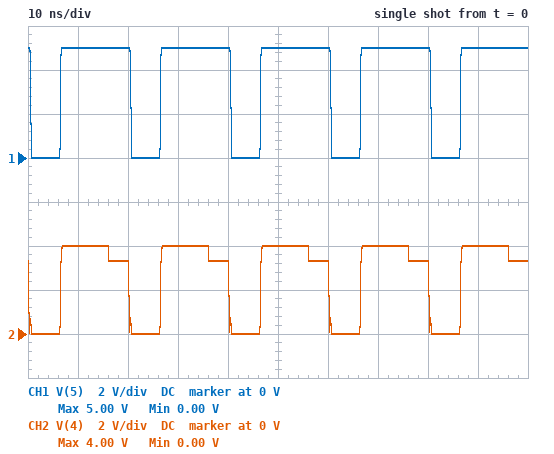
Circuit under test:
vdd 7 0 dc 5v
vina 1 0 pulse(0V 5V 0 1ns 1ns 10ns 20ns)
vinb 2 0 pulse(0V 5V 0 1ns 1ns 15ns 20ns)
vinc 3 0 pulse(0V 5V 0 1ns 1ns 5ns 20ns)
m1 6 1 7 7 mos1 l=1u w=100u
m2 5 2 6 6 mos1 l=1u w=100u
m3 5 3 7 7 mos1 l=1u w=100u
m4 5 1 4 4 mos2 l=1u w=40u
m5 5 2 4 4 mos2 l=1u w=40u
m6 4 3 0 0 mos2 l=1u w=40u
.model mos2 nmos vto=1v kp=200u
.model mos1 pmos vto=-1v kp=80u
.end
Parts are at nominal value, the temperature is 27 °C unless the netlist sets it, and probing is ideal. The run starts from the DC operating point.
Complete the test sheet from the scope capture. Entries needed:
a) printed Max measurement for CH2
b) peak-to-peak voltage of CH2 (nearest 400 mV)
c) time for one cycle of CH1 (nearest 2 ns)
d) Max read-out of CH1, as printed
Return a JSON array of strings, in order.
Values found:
["4.00 V", "4.0 V", "20 ns", "5.00 V"]
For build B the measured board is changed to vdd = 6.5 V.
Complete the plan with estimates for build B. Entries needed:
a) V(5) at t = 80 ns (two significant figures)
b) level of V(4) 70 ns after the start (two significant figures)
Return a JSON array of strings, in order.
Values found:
["6.5 V", "4.3 V"]
